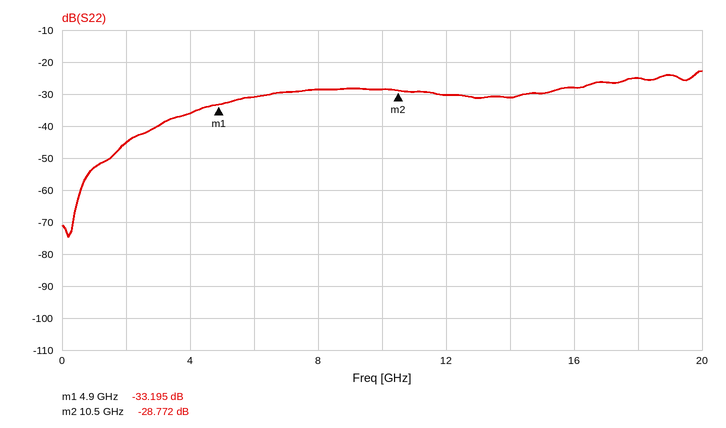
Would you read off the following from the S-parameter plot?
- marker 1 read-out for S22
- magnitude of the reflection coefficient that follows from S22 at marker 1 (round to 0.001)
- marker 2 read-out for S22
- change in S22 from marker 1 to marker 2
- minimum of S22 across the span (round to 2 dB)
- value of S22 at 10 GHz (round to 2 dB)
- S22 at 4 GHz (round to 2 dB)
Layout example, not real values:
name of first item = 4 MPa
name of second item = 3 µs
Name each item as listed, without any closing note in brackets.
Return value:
marker 1 read-out for S22 = -33.195 dB
magnitude of the reflection coefficient that follows from S22 at marker 1 = 0.022
marker 2 read-out for S22 = -28.772 dB
change in S22 from marker 1 to marker 2 = 4.423 dB
minimum of S22 across the span = -74 dB
value of S22 at 10 GHz = -28 dB
S22 at 4 GHz = -36 dB
